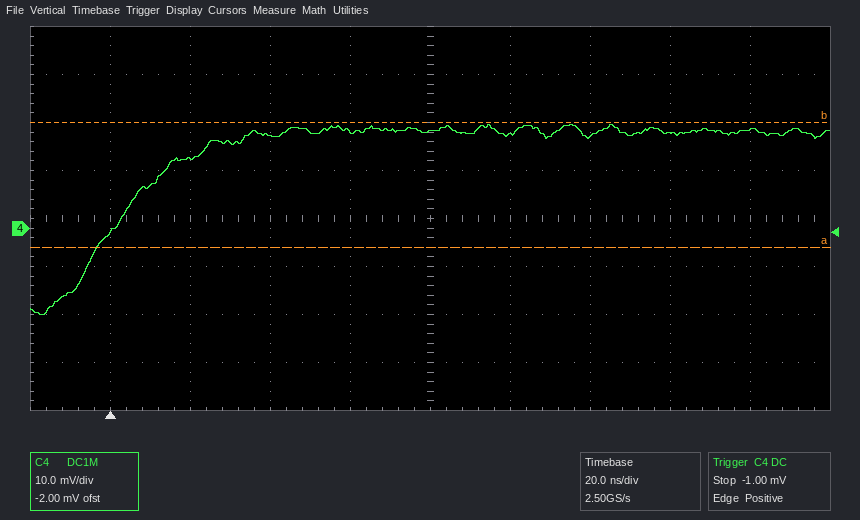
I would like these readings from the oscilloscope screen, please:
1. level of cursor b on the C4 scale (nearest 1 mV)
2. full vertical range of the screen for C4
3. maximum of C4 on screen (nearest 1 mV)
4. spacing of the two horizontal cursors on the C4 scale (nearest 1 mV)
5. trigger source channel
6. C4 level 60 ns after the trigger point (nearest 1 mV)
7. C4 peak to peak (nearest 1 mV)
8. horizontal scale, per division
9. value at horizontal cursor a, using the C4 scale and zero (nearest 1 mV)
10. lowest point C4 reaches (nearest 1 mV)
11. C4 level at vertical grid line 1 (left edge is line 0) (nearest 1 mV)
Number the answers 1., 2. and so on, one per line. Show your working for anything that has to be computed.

1. 22 mV
2. 80 mV
3. 22 mV
4. 26 mV
5. C4
6. 20 mV
7. 22 mV − (-18 mV) = 40 mV
8. 20 ns
9. -4 mV
10. -18 mV
11. -1 mV
